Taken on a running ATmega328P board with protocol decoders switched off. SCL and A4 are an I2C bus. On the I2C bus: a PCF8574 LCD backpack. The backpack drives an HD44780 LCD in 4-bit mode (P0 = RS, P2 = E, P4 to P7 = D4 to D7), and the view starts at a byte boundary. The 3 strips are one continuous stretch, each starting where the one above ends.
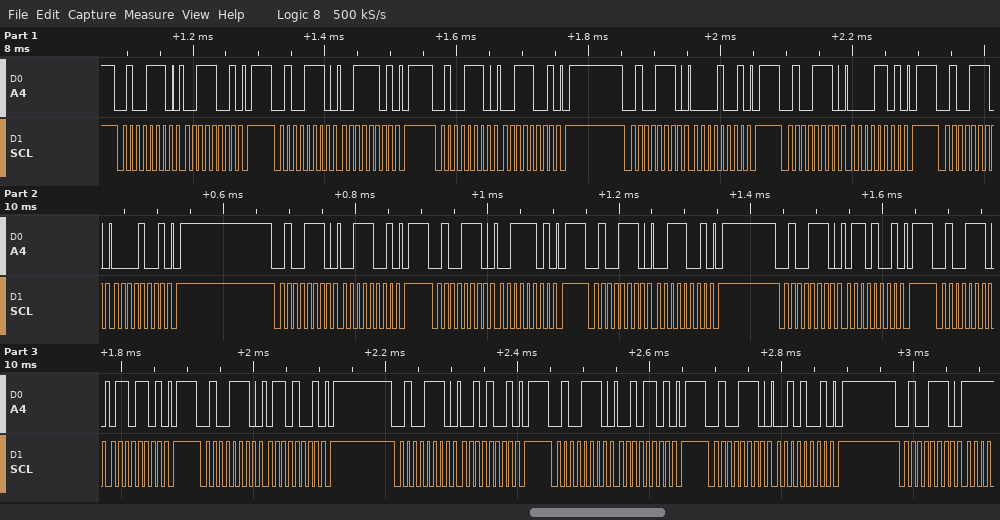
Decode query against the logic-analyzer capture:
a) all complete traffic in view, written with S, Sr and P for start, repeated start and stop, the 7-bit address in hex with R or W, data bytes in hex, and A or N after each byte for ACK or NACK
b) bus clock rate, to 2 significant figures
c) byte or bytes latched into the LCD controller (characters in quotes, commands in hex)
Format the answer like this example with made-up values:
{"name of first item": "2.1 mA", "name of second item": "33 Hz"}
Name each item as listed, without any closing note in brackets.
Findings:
{"all complete traffic in view, written with S, Sr and P for start, repeated start and stop, the 7-bit address in hex with R or W, data bytes in hex, and A or N after each byte for ACK or NACK": "S 27W A 39 A P S 27W A 3D A P S 27W A 39 A P S 27W A 09 A P S 27W A 0D A P S 27W A 09 A P S 27W A 39 A P S 27W A 3D A P S 27W A 39 A P S 27W A 69 A P S 27W A 6D A P S 27W A 69 A P S 27W A 29 A P S 27W A 2D A P S 27W A 29 A P S 27W A", "bus clock rate, to 2 significant figures": "100 kHz", "byte or bytes latched into the LCD controller": "'0' '6'"}
